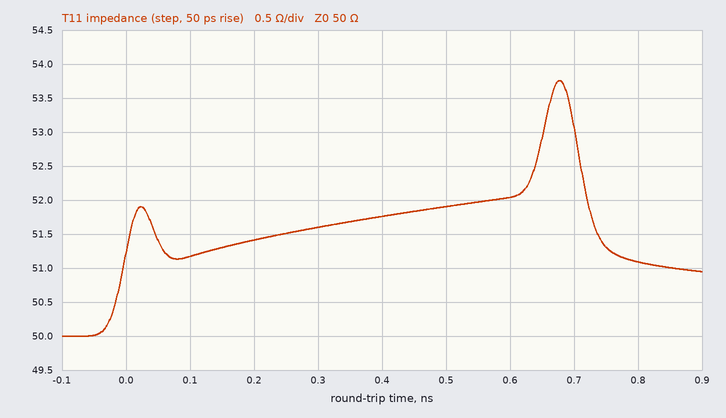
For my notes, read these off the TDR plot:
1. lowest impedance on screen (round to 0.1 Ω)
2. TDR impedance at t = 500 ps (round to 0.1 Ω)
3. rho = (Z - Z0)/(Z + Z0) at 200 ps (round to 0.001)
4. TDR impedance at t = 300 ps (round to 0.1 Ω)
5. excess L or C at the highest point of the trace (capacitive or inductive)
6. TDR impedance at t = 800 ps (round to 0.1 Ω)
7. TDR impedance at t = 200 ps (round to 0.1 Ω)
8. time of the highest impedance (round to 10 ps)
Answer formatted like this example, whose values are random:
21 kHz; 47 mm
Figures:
50.0 Ω; 51.9 Ω; +0.014; 51.6 Ω; inductive; 51.1 Ω; 51.4 Ω; 680 ps
